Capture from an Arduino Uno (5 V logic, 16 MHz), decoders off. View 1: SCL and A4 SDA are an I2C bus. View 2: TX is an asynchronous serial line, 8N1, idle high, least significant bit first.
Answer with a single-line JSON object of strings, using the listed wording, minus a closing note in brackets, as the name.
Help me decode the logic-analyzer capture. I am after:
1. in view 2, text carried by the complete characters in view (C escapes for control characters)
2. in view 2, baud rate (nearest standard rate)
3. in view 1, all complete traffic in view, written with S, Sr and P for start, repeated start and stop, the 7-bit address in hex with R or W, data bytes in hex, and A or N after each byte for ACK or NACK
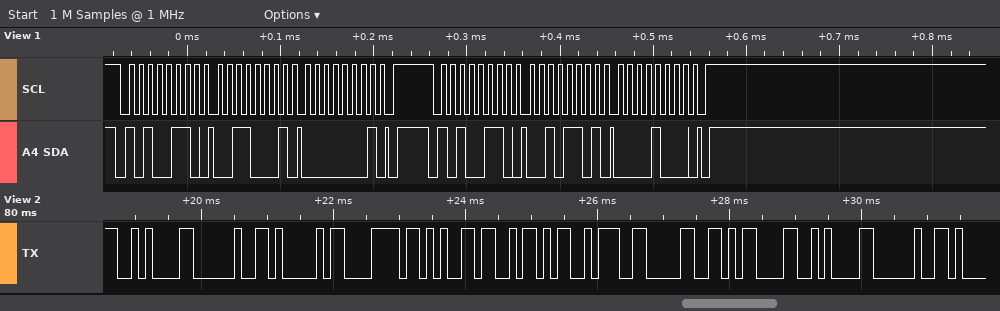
{"in view 2, text carried by the complete characters in view": "\"\\n AxeZ:0\\r\\n \"", "in view 2, baud rate": "9600 baud", "in view 1, all complete traffic in view, written with S, Sr and P for start, repeated start and stop, the 7-bit address in hex with R or W, data bytes in hex, and A or N after each byte for ACK or NACK": "S 53W A 31 A 01 A P S 53W A 2D A 08 A P"}
